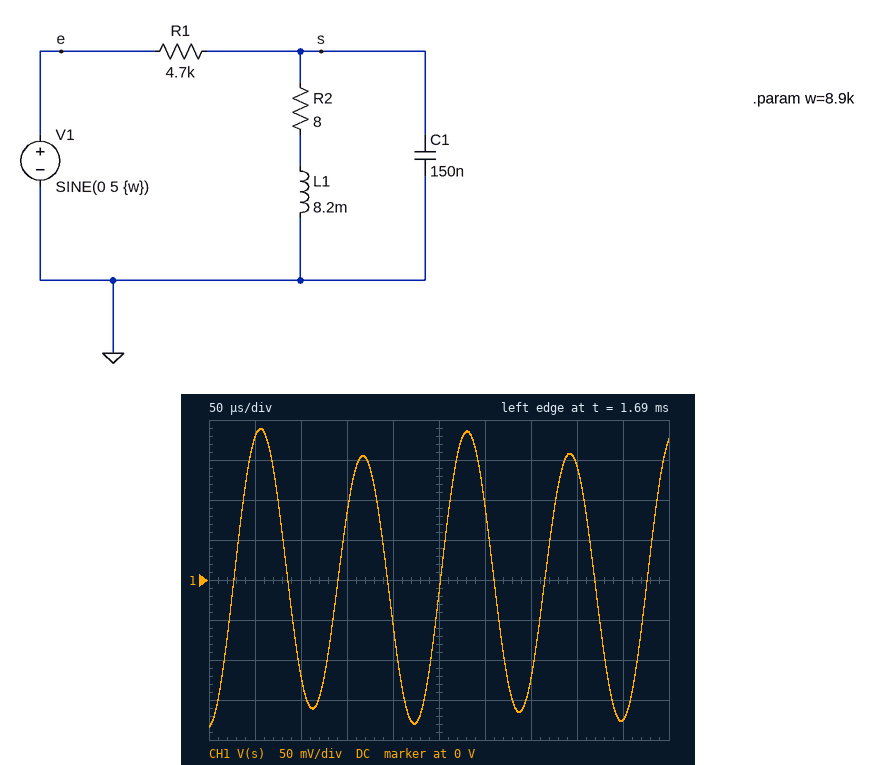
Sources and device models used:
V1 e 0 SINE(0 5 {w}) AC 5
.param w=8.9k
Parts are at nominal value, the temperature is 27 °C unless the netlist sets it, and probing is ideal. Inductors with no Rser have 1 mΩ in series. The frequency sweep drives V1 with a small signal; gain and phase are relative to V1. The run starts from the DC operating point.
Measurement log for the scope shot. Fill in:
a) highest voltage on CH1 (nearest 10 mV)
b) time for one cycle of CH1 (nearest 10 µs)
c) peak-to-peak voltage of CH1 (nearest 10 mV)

190 mV
110 µs
370 mV
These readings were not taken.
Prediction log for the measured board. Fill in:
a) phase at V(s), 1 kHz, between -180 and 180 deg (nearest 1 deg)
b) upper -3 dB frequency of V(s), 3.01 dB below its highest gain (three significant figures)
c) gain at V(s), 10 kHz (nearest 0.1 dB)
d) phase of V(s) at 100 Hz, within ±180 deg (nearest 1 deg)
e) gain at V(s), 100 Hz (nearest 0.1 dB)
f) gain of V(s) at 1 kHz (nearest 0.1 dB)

80 deg
4.74 kHz
-30.9 dB
33 deg
-53.9 dB
-38.7 dB
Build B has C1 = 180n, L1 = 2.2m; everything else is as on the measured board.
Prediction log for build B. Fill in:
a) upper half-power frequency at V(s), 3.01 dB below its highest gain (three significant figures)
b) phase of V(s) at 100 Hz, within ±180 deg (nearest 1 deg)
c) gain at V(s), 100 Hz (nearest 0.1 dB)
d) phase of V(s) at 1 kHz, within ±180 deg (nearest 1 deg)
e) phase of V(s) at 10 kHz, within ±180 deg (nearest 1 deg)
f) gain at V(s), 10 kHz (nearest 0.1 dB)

8.40 kHz
10 deg
-55.3 dB
59 deg
-81 deg
-25.8 dB
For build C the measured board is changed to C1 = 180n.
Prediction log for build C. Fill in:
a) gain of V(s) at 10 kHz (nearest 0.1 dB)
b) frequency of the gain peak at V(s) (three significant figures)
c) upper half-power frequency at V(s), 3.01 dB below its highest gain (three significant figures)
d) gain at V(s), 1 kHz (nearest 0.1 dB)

-32.9 dB
4.15 kHz
4.32 kHz
-38.6 dB
